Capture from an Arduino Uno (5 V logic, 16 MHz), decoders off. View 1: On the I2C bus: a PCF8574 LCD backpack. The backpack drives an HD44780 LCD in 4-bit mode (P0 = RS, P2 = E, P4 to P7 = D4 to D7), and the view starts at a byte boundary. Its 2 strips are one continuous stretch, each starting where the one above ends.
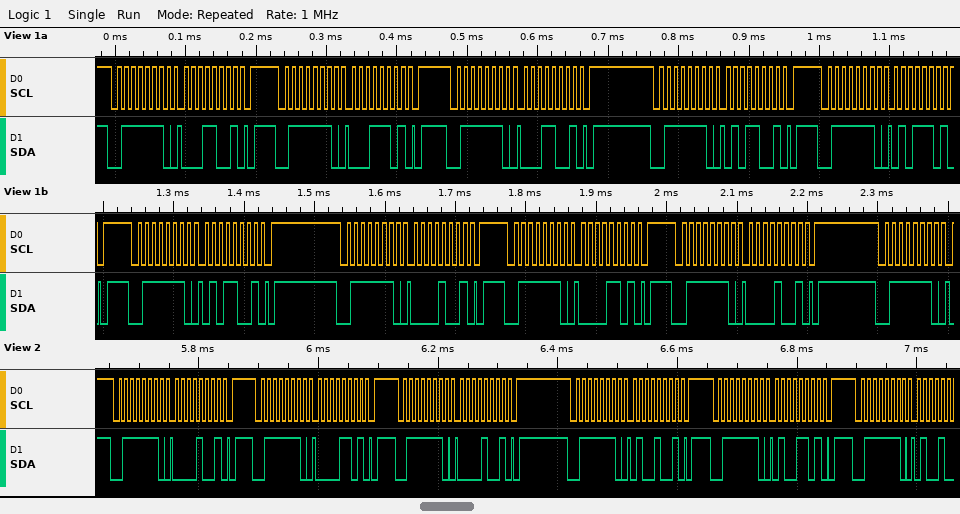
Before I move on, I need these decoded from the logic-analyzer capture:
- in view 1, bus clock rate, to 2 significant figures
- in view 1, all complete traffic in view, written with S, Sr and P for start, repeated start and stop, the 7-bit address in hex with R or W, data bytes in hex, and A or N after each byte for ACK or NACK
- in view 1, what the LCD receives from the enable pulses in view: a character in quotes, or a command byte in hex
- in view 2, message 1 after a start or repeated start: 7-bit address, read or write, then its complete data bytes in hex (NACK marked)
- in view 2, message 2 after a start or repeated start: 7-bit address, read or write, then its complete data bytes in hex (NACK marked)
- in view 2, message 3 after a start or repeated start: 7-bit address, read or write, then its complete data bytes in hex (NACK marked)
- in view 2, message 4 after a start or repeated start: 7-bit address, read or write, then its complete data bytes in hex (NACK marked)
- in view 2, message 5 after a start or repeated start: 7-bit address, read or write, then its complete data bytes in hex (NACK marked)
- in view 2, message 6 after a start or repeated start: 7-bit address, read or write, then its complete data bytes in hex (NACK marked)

100 kHz
S 3FW A 19 A P S 3FW A 1D A P S 3FW A 19 A P S 3FW A 59 A P S 3FW A 5D A P S 3FW A 59 A P S 3FW A 09 A P S 3FW A 0D A P S 3FW A 09 A P S 3FW A
data 0x15
0x3F write: 09
0x3F write: 0D
0x3F write: 09
0x3F write: 49
0x3F write: 4D
0x3F write
